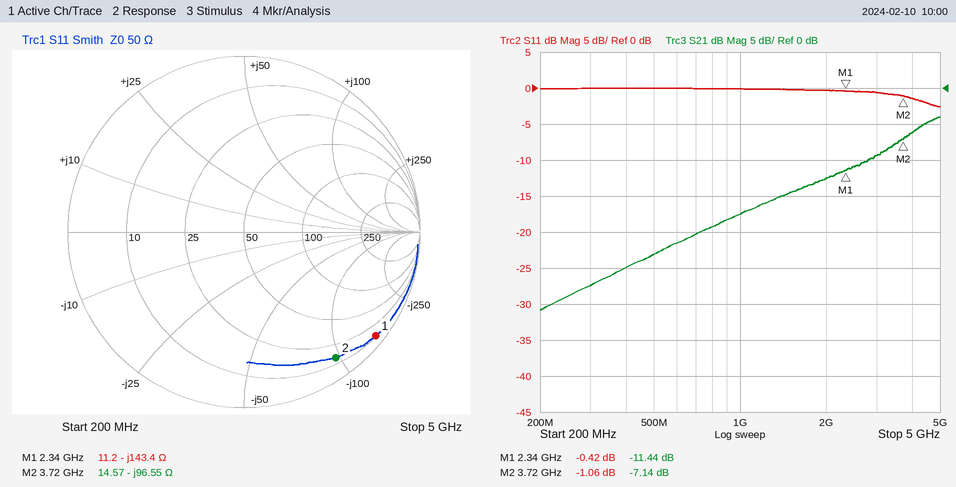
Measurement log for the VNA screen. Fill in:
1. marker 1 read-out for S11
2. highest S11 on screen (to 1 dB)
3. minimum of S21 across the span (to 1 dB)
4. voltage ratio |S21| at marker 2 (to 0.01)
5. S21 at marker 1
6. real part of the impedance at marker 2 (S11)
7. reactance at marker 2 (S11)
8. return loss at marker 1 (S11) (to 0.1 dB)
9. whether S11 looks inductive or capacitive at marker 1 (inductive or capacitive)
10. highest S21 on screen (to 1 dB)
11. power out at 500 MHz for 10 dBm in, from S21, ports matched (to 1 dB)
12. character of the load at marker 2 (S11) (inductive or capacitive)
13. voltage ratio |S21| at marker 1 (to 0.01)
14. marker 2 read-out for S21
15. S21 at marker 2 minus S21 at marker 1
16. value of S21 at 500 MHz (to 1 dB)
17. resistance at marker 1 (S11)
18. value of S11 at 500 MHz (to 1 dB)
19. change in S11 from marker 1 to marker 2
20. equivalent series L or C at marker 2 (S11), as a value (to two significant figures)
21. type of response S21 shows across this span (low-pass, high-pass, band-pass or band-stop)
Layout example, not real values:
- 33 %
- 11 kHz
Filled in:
- -0.42 dB
- 0 dB
- -31 dB
- 0.44
- -11.44 dB
- 14.57 Ω
- -96.55 Ω
- 0.4 dB
- capacitive
- -4 dB
- -13 dBm
- capacitive
- 0.27
- -7.14 dB
- 4.30 dB
- -23 dB
- 11.2 Ω
- 0 dB
- -0.64 dB
- 440 fF
- high-pass
